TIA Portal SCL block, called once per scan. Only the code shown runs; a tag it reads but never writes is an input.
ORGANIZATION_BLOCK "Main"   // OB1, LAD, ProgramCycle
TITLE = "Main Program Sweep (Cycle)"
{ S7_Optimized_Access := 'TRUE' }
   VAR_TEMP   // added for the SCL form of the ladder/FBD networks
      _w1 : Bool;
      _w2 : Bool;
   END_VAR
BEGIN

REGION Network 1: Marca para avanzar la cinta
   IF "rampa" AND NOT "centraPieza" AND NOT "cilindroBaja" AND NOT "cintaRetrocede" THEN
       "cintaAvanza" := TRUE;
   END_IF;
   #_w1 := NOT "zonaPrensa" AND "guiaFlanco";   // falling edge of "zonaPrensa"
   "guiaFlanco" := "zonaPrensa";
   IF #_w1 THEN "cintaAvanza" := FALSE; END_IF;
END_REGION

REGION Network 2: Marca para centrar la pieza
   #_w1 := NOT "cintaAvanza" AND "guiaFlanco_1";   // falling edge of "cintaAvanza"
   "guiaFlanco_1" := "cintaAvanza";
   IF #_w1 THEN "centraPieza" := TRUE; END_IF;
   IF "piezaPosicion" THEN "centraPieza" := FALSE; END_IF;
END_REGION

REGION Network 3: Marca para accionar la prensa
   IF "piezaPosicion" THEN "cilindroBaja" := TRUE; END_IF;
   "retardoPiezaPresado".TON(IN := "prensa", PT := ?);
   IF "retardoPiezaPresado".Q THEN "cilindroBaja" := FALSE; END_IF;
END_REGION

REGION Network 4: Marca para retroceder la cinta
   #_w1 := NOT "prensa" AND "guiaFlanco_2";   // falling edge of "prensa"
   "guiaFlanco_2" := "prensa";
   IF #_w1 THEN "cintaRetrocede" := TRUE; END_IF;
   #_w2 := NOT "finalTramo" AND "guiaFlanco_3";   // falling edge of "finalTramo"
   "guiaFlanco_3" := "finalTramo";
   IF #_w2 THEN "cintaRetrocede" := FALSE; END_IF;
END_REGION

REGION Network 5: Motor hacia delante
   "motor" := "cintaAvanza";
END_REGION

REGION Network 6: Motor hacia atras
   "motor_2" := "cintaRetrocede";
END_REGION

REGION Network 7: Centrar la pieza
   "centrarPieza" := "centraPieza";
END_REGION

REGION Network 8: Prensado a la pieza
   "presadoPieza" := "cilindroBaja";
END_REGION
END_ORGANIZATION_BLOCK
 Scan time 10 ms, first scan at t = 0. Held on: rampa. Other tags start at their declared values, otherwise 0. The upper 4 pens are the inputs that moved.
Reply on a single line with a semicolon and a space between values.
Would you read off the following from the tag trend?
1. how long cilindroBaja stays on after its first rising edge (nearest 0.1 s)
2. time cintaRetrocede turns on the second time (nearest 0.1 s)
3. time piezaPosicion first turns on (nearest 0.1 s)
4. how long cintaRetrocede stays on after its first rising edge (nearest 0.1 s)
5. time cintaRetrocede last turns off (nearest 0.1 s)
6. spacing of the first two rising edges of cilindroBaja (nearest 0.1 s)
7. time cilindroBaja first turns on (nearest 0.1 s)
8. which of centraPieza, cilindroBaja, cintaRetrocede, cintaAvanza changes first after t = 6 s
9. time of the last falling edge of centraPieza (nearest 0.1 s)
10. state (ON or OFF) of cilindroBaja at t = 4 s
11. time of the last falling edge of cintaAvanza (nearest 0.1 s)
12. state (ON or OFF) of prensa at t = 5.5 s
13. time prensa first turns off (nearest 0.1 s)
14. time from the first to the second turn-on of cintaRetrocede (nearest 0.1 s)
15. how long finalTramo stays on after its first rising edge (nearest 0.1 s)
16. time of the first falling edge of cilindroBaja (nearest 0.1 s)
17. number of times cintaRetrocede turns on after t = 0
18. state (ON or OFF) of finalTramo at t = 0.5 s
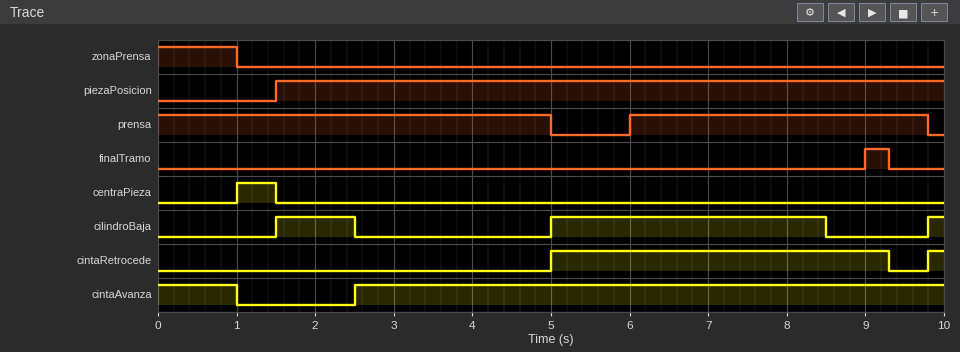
1.0 s; 9.8 s; 1.5 s; 4.3 s; 9.3 s; 3.5 s; 1.5 s; cilindroBaja; 1.5 s; OFF; 1.0 s; OFF; 5.0 s; 4.8 s; 0.3 s; 2.5 s; 2; OFF
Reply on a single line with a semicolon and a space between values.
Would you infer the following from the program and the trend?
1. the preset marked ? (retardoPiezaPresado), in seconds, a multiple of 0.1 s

2.5 s
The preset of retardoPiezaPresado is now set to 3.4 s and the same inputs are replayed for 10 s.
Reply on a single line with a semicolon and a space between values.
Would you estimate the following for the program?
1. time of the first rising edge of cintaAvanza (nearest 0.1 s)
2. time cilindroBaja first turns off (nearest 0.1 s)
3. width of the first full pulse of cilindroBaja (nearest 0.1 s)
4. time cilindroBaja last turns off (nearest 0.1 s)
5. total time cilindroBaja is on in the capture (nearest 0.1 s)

3.4 s; 3.4 s; 1.9 s; 9.4 s; 6.5 s
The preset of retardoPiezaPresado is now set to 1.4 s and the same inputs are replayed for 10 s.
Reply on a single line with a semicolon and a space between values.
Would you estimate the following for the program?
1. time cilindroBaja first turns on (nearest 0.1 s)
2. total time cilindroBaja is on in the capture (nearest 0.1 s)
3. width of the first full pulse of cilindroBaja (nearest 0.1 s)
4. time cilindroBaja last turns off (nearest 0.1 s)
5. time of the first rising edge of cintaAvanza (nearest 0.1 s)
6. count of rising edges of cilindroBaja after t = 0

5.0 s; 2.6 s; 2.4 s; 7.4 s; 1.5 s; 2
